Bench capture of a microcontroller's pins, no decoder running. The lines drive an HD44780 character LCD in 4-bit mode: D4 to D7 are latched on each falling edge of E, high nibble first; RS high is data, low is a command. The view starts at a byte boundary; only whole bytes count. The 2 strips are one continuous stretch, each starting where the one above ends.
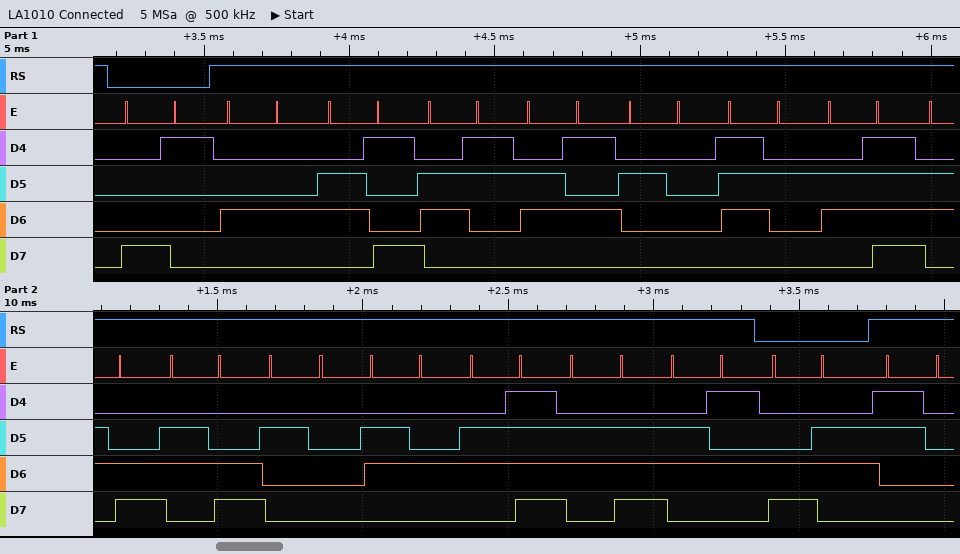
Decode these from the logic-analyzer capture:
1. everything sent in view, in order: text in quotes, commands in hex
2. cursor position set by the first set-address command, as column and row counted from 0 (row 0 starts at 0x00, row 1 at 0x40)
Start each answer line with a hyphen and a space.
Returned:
- 0x81 "Dice roll done" 0xC6 "0"
- column 1, row 0
